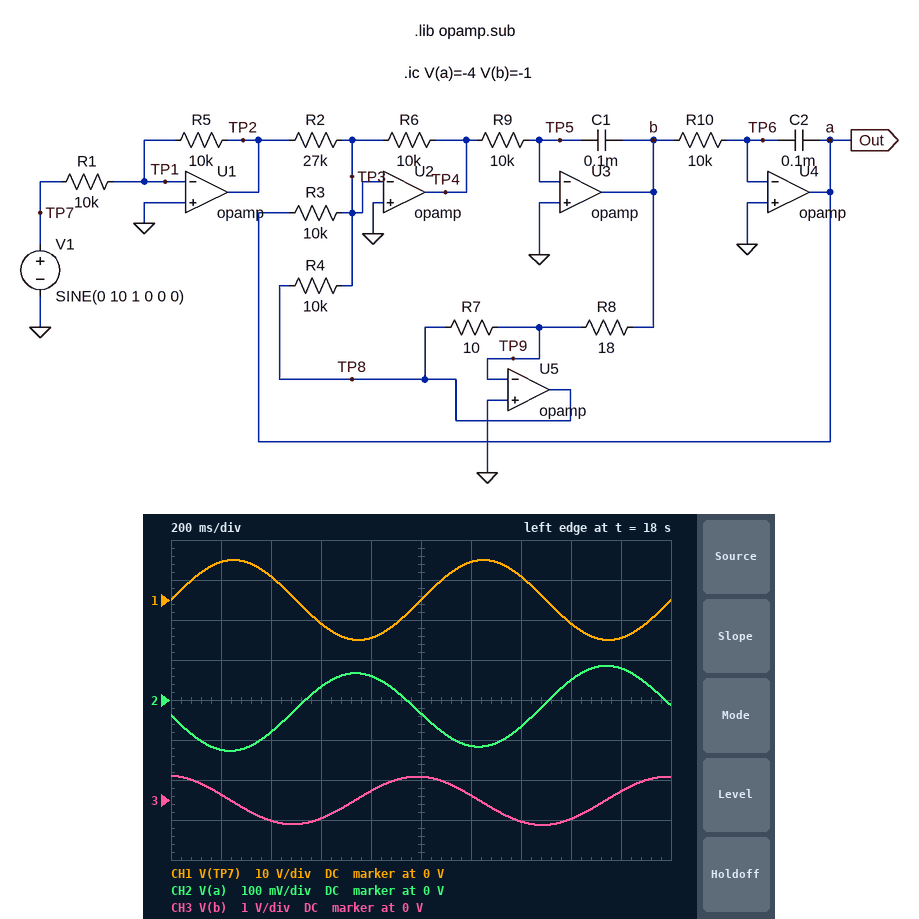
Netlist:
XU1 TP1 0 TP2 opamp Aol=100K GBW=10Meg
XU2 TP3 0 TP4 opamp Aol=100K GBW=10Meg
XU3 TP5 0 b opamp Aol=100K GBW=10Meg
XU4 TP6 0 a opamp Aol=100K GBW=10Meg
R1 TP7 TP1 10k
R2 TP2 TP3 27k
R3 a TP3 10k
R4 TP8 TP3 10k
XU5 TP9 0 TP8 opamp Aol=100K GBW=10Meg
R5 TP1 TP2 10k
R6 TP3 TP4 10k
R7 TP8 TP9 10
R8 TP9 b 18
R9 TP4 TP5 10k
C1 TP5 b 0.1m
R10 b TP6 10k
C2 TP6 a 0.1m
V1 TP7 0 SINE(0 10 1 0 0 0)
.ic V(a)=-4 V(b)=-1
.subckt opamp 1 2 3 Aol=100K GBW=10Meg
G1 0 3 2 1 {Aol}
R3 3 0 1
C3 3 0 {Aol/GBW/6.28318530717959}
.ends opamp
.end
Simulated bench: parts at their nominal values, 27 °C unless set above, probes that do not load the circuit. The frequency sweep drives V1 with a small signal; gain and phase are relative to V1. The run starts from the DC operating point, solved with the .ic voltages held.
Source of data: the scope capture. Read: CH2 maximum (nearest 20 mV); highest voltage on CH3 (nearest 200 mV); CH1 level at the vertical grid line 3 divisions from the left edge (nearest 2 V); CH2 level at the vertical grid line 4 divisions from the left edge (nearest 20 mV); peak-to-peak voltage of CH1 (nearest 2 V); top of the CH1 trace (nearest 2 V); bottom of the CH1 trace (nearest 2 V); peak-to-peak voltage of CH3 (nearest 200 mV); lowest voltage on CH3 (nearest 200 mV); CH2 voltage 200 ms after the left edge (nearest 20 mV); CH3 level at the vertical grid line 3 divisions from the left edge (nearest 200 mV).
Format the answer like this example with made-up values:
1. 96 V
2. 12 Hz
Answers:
1. 80 mV
2. 600 mV
3. -6 V
4. 60 mV
5. 20 V
6. 10 V
7. -10 V
8. 1.2 V
9. -600 mV
10. -120 mV
11. -400 mV
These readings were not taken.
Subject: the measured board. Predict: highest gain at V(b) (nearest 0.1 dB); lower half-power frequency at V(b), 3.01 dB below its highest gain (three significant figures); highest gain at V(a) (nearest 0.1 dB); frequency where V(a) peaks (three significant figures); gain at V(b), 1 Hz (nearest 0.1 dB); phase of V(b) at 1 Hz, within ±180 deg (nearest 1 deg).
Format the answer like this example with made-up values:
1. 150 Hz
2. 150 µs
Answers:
1. -3.5 dB
2. 121 mHz
3. -3.2 dB
4. 146 mHz
5. -24.4 dB
6. 95 deg
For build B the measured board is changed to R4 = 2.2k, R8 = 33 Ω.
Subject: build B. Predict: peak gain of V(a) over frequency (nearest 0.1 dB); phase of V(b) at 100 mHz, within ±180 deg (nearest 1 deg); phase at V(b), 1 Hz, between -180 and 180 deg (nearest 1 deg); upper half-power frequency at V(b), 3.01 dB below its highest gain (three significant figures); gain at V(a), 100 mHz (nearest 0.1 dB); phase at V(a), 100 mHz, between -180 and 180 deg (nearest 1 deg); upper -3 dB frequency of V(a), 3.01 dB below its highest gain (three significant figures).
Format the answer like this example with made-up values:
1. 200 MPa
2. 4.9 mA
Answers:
1. -8.6 dB
2. -145 deg
3. 103 deg
4. 303 mHz
5. -9.1 dB
6. -55 deg
7. 163 mHz
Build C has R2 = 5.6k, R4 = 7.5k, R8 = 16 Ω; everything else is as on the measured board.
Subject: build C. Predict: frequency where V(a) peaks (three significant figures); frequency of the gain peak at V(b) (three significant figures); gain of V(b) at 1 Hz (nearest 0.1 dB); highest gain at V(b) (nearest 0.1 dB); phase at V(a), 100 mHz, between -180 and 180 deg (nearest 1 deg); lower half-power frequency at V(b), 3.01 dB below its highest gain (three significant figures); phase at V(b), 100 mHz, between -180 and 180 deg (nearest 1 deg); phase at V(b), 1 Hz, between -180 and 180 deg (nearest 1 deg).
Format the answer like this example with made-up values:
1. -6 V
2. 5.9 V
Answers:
1. 129 mHz
2. 159 mHz
3. -10.8 dB
4. 6.6 dB
5. -41 deg
6. 106 mHz
7. -131 deg
8. 98 deg
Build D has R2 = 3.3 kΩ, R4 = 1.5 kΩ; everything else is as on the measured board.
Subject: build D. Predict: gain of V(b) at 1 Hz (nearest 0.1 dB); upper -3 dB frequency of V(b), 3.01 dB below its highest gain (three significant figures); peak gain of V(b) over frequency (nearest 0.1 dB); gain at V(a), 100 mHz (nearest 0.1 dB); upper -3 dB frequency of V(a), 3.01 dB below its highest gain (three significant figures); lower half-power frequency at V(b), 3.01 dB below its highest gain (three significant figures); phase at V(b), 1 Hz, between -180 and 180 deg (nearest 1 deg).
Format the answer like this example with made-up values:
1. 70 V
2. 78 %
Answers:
1. -7.5 dB
2. 630 mHz
3. -1.7 dB
4. 2.0 dB
5. 46.3 mHz
6. 40.2 mHz
7. 121 deg
